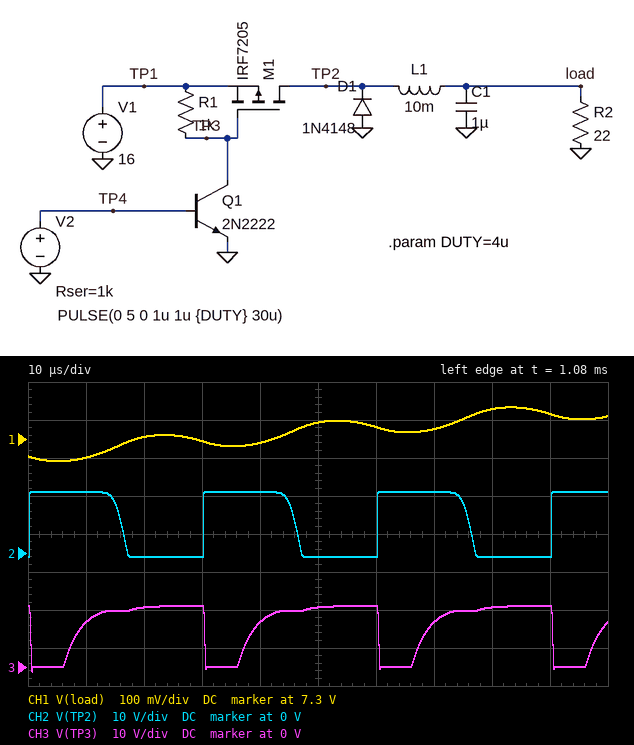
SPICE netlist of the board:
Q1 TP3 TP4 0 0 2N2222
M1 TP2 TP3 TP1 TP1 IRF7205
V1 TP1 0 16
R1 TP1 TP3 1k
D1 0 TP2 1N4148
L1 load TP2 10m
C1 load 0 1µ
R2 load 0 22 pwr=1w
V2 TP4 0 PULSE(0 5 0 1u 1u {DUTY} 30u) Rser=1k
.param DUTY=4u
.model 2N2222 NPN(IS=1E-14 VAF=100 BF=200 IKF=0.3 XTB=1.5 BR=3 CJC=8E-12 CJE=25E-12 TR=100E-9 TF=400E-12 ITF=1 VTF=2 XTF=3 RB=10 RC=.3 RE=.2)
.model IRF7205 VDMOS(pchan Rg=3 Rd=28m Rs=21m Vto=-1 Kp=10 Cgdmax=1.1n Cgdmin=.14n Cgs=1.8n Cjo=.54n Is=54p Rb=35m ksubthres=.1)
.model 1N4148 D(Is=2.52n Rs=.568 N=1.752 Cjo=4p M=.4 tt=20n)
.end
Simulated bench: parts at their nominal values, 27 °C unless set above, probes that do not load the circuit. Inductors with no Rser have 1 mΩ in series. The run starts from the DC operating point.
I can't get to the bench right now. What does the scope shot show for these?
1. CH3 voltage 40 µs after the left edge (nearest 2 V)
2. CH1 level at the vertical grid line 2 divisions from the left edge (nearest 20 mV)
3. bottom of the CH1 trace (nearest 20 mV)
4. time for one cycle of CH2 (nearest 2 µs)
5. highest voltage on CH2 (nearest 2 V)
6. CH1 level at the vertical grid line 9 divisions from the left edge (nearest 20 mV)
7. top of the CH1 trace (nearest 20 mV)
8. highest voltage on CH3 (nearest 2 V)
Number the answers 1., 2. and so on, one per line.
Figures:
1. 12 V
2. 7.30 V
3. 7.24 V
4. 30 µs
5. 16 V
6. 7.36 V
7. 7.38 V
8. 16 V
